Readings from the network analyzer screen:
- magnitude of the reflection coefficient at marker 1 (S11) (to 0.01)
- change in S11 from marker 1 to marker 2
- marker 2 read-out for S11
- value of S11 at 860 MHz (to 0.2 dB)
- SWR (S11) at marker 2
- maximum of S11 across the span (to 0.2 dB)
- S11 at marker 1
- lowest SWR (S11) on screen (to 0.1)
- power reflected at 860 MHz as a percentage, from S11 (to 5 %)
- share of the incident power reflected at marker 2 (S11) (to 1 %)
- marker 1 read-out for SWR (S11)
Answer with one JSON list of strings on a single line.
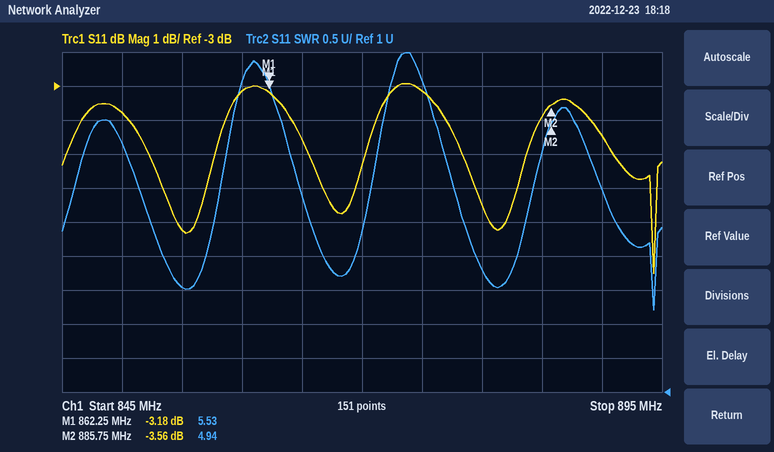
["0.69", "-0.38 dB", "-3.56 dB", "-3.2 dB", "4.94", "-3.0 dB", "-3.18 dB", "2.2", "50 %", "44 %", "5.53"]
